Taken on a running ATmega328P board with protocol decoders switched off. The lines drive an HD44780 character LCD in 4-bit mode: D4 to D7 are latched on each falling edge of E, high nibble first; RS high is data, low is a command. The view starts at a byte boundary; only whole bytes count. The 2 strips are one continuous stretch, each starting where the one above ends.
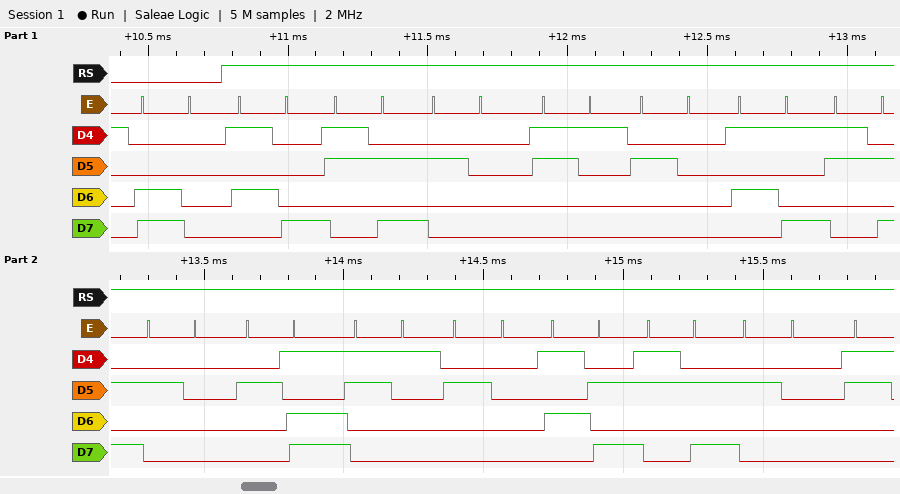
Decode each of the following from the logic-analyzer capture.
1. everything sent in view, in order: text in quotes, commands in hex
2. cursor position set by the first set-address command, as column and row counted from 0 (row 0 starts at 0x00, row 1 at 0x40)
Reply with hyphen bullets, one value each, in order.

- 0xC0 "X: 1 Y: -1 Z: "
- column 0, row 1
